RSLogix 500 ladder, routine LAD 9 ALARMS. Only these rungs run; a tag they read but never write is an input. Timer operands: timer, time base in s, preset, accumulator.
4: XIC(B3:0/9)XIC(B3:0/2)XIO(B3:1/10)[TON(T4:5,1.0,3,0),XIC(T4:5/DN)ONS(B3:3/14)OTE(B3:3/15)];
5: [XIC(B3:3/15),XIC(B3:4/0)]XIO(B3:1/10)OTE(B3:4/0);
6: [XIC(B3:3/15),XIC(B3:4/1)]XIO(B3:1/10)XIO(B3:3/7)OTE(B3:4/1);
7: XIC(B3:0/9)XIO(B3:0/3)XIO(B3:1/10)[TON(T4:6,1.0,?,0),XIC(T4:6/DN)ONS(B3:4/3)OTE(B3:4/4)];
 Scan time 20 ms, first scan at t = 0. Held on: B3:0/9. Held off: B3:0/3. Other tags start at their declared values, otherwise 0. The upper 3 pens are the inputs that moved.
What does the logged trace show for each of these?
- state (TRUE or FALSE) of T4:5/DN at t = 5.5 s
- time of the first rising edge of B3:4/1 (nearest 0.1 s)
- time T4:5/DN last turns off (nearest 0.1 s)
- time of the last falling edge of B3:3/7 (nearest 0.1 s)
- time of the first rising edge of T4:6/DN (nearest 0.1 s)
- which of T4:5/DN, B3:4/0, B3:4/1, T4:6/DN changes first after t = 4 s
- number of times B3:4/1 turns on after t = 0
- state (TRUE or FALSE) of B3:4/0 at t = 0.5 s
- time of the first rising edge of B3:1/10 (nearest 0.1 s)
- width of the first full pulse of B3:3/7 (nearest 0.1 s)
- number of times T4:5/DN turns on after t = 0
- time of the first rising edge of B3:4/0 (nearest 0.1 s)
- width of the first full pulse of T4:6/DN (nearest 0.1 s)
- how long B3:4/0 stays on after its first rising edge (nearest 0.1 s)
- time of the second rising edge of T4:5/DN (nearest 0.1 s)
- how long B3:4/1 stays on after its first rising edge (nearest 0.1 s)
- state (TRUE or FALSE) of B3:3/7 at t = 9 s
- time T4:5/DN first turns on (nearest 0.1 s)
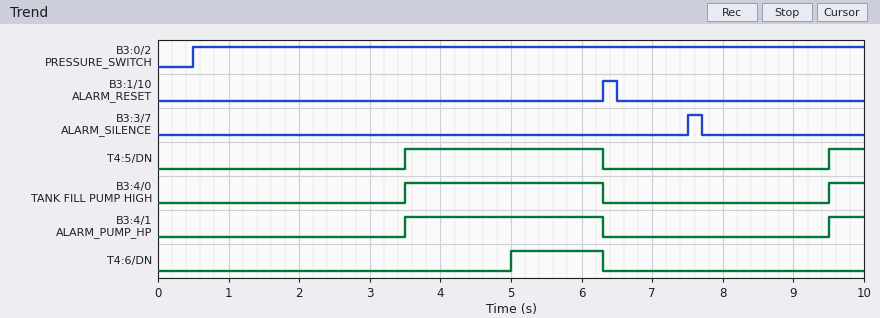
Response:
TRUE
3.5 s
6.3 s
7.7 s
5.0 s
T4:6/DN
2
FALSE
6.3 s
0.2 s
2
3.5 s
1.3 s
2.8 s
9.5 s
2.8 s
FALSE
3.5 s
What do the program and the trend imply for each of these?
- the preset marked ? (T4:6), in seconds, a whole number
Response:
5 s
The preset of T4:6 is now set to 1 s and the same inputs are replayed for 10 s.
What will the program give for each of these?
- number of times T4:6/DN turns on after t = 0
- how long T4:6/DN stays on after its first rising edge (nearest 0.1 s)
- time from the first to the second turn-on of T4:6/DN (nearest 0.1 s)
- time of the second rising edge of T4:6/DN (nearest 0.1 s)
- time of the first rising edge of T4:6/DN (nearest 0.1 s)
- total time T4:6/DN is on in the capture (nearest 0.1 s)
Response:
2
5.3 s
6.5 s
7.5 s
1.0 s
7.8 s
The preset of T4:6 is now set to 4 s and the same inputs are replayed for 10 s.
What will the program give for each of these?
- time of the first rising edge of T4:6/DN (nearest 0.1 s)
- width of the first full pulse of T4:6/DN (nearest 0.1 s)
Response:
4.0 s
2.3 s
